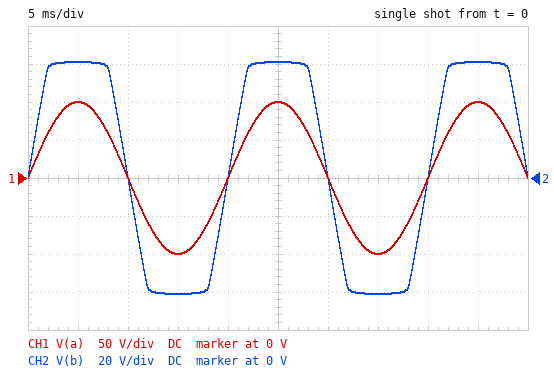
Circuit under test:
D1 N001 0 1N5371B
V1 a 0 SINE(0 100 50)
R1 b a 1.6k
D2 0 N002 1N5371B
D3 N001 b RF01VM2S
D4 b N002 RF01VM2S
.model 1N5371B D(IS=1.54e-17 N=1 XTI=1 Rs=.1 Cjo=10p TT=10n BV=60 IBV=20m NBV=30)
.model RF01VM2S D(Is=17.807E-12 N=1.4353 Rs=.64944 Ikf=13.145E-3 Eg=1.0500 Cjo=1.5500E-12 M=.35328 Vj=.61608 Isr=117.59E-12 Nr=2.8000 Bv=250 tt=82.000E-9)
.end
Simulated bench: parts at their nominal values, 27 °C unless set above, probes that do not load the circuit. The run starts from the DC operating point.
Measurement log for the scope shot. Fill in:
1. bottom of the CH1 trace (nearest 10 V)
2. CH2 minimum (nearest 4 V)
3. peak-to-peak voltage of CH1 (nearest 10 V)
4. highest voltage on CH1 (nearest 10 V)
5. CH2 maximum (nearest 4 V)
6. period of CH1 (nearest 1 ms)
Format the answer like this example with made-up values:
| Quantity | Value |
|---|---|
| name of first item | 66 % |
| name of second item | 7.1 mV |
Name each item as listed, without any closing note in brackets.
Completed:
| Quantity | Value |
|---|---|
| bottom of the CH1 trace | -100 V |
| CH2 minimum | -60 V |
| peak-to-peak voltage of CH1 | 200 V |
| highest voltage on CH1 | 100 V |
| CH2 maximum | 60 V |
| period of CH1 | 20 ms |
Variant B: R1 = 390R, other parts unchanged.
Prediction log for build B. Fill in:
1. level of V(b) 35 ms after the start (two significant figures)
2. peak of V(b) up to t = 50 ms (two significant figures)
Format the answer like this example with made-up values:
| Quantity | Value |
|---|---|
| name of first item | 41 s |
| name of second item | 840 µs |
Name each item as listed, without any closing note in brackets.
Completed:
| Quantity | Value |
|---|---|
| level of V(b) 35 ms after the start | -62 V |
| peak of V(b) up to t = 50 ms | 62 V |
